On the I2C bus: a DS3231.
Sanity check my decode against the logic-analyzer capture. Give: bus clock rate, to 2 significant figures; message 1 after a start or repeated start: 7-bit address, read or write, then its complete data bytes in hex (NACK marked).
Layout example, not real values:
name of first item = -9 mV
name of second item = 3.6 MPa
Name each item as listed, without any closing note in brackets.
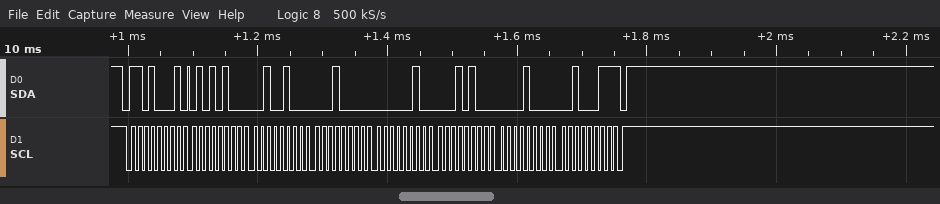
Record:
bus clock rate, to 2 significant figures = 100 kHz
message 1 after a start or repeated start: 7-bit address, read or write, then its complete data bytes in hex = 0x68 read: 54 24 10 02 14 08 23 NACK
